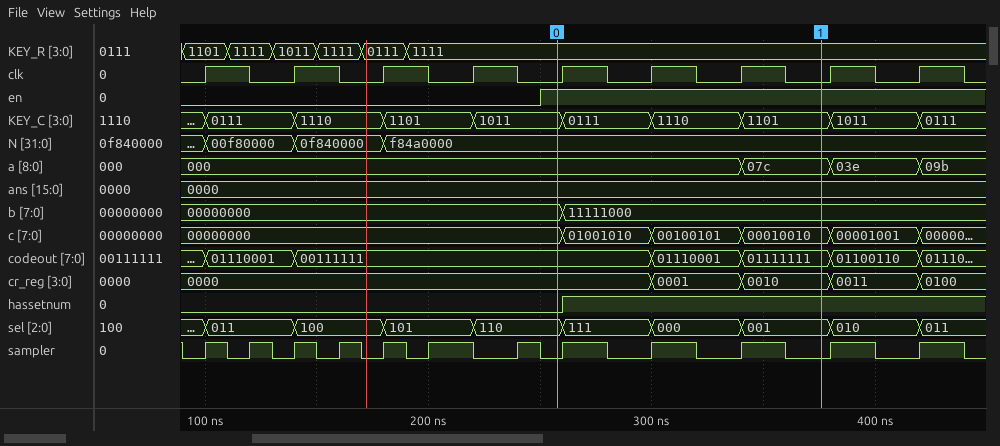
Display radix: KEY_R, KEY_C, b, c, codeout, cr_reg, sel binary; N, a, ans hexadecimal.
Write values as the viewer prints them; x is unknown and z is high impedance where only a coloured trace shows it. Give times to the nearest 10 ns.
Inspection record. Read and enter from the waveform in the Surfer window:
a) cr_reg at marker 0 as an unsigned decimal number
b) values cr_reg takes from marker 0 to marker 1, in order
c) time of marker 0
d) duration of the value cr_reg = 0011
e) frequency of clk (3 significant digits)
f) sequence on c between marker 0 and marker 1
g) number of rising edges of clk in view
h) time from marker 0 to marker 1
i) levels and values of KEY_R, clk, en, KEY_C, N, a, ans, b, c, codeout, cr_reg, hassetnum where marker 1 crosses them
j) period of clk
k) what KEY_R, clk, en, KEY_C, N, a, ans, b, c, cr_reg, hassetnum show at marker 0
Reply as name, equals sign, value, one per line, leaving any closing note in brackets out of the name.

cr_reg at marker 0 as an unsigned decimal number = 0
values cr_reg takes from marker 0 to marker 1, in order = 0000, 0001, 0010
time of marker 0 = 260 ns
duration of the value cr_reg = 0011 = 40 ns
frequency of clk = 25.0 MHz
sequence on c between marker 0 and marker 1 = 00000000, 01001010, 00100101, 00010010
number of rising edges of clk in view = 9
time from marker 0 to marker 1 = 120 ns
levels and values of KEY_R, clk, en, KEY_C, N, a, ans, b, c, codeout, cr_reg, hassetnum where marker 1 crosses them = KEY_R=1111, clk=0, en=1, KEY_C=1101, N=f84a0000, a=07c, ans=0000, b=11111000, c=00010010, codeout=01111111, cr_reg=0010, hassetnum=1
period of clk = 40 ns
what KEY_R, clk, en, KEY_C, N, a, ans, b, c, cr_reg, hassetnum show at marker 0 = KEY_R=1111, clk=0, en=1, KEY_C=1011, N=f84a0000, a=000, ans=0000, b=00000000, c=00000000, cr_reg=0000, hassetnum=0
